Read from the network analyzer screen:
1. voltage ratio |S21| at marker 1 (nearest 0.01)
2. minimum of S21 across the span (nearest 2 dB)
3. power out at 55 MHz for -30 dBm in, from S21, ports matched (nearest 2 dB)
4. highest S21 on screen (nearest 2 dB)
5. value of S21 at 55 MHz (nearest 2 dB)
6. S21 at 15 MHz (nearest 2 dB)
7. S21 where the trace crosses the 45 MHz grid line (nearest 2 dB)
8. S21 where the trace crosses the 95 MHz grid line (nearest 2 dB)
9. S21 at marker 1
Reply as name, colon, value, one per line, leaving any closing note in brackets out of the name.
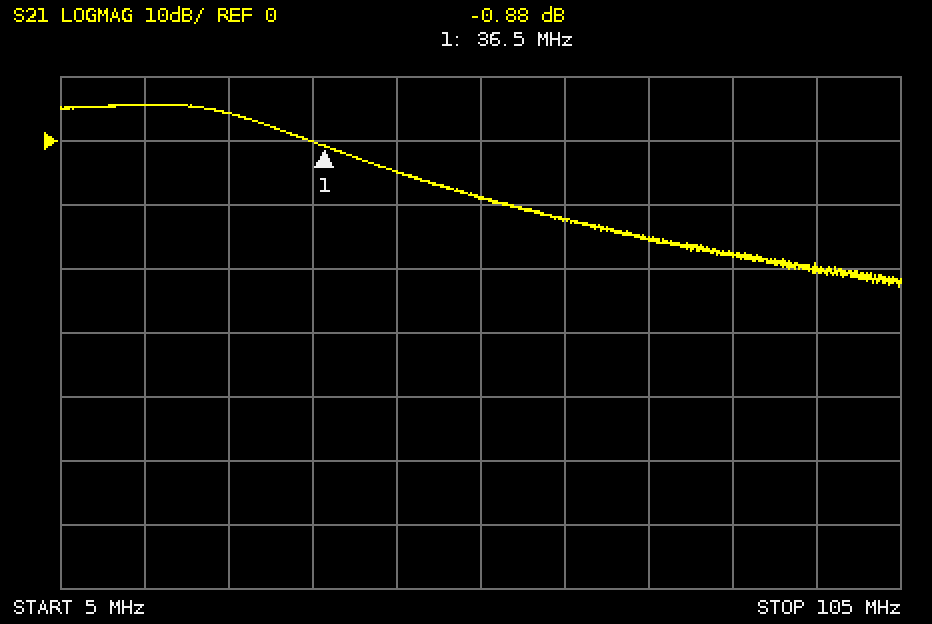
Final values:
voltage ratio |S21| at marker 1: 0.90
minimum of S21 across the span: -22 dB
power out at 55 MHz for -30 dBm in, from S21, ports matched: -38 dBm
highest S21 on screen: 6 dB
value of S21 at 55 MHz: -8 dB
S21 at 15 MHz: 6 dB
S21 where the trace crosses the 45 MHz grid line: -4 dB
S21 where the trace crosses the 95 MHz grid line: -20 dB
S21 at marker 1: -0.88 dB
